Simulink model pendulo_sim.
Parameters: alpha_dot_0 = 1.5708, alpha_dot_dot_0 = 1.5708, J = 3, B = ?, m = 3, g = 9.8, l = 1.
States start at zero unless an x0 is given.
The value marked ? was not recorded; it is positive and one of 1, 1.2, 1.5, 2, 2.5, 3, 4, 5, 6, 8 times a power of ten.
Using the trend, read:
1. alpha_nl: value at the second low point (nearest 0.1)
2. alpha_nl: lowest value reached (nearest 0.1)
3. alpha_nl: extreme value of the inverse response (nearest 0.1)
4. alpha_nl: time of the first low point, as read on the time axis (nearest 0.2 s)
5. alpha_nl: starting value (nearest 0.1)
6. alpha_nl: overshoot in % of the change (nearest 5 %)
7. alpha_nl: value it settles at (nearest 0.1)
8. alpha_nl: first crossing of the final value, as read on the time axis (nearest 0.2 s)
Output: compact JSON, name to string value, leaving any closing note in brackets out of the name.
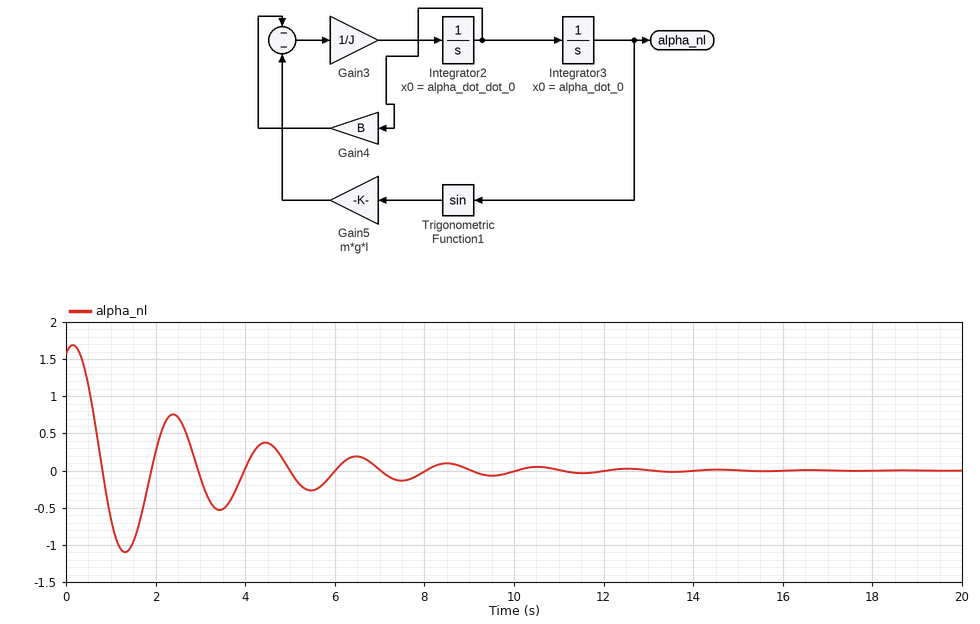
{"alpha_nl: value at the second low point": "-0.5", "alpha_nl: lowest value reached": "-1.1", "alpha_nl: extreme value of the inverse response": "1.7", "alpha_nl: time of the first low point, as read on the time axis": "1.4 s", "alpha_nl: starting value": "1.6", "alpha_nl: overshoot in % of the change": "70 %", "alpha_nl: value it settles at": "0.0", "alpha_nl: first crossing of the final value, as read on the time axis": "0.8 s"}
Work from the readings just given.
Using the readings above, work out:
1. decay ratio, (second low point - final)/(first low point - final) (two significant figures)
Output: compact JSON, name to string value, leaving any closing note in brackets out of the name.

{"decay ratio, (second low point - final)/(first low point - final)": "0.45"}
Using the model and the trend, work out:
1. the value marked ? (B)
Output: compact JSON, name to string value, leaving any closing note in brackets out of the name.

{"the value marked ?": "2"}
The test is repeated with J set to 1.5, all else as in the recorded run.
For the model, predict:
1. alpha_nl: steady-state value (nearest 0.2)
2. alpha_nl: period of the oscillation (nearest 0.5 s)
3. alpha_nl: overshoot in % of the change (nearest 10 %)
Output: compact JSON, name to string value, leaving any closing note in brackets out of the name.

{"alpha_nl: steady-state value": "0.0", "alpha_nl: period of the oscillation": "1.5 s", "alpha_nl: overshoot in % of the change": "60 %"}
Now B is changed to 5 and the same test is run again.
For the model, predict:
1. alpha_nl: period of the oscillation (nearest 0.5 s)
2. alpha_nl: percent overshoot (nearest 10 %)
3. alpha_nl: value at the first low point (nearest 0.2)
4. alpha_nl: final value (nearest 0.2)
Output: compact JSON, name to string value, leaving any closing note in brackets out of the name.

{"alpha_nl: period of the oscillation": "2.0 s", "alpha_nl: percent overshoot": "40 %", "alpha_nl: value at the first low point": "-0.6", "alpha_nl: final value": "0.0"}
